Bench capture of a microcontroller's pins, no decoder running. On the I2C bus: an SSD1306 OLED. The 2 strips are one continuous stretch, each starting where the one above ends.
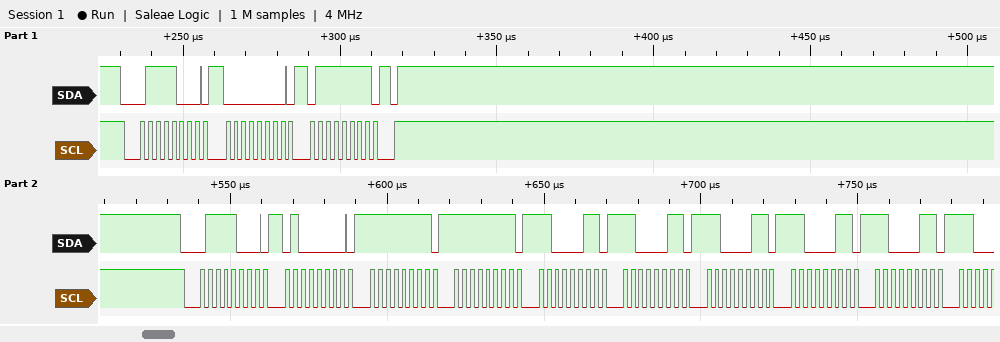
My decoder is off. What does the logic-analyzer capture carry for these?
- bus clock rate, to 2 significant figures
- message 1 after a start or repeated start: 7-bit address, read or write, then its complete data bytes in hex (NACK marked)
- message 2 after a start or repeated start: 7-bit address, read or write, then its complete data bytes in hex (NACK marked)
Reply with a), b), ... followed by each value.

a) 400 kHz
b) 0x3C write: 00 7F
c) 0x3C write: 40 FF FF C3 C3 C3 C3 C3
